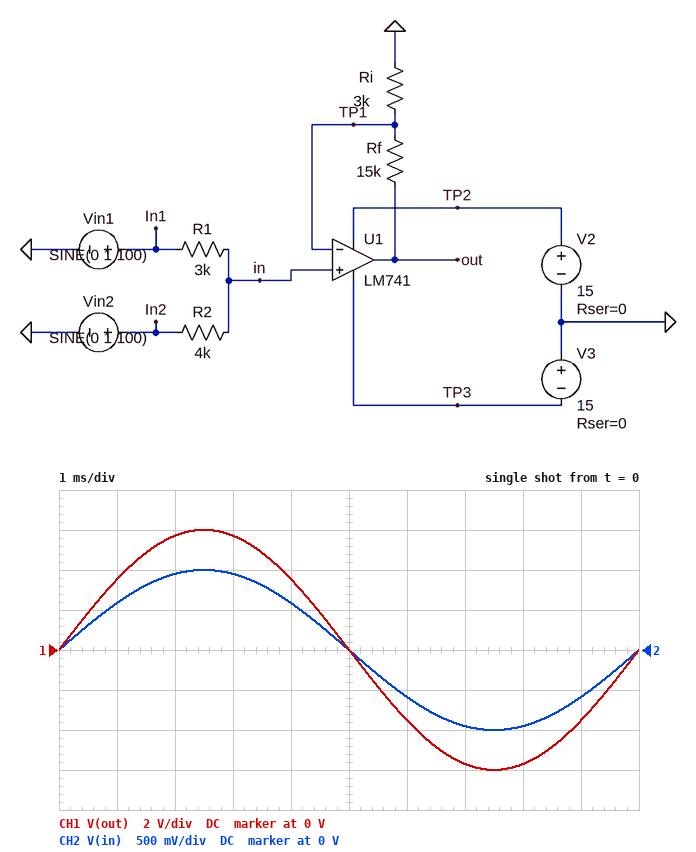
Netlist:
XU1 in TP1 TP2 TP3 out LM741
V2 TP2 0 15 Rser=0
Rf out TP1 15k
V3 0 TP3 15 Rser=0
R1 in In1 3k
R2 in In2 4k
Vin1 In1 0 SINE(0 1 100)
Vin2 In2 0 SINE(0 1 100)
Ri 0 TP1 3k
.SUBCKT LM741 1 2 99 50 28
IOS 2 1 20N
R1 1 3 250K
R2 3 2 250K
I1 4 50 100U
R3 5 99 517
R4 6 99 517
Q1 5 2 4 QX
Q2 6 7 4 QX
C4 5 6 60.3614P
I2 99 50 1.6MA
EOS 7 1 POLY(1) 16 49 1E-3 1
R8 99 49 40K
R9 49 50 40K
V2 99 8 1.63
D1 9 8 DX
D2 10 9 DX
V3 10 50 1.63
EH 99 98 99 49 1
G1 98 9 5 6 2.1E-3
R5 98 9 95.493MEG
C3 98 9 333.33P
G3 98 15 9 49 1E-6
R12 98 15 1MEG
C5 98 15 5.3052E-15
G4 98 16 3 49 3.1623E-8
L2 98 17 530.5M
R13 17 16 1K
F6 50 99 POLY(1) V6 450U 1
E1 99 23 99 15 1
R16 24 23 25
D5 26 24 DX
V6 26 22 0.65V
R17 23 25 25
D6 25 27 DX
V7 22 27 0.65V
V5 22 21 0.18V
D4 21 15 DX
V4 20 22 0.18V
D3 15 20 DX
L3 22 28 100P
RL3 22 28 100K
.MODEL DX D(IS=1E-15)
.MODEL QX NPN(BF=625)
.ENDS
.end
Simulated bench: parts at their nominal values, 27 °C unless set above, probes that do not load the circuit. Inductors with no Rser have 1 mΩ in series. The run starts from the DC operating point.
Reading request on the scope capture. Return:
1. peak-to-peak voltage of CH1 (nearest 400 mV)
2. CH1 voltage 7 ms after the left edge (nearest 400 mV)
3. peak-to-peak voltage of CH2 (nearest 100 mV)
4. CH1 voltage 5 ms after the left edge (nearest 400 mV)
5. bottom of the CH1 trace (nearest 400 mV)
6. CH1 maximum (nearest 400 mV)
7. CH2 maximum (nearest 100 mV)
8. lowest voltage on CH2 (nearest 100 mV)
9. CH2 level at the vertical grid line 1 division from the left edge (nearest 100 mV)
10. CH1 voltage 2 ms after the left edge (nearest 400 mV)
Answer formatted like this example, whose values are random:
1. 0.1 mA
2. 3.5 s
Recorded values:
1. 12.0 V
2. -5.6 V
3. 2.0 V
4. 0 V
5. -6.0 V
6. 6.0 V
7. 1.0 V
8. -1.0 V
9. 600 mV
10. 5.6 V
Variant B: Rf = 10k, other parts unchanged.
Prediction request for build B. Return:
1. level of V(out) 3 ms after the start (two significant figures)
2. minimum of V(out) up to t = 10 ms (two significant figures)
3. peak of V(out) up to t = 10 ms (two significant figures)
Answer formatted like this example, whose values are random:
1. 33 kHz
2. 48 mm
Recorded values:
1. 4.1 V
2. -4.3 V
3. 4.3 V
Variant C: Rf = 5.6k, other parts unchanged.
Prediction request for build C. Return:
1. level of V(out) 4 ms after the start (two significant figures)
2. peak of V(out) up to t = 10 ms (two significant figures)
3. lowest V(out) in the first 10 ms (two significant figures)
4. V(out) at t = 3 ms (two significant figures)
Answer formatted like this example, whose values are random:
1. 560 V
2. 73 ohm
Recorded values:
1. 1.7 V
2. 2.9 V
3. -2.9 V
4. 2.7 V
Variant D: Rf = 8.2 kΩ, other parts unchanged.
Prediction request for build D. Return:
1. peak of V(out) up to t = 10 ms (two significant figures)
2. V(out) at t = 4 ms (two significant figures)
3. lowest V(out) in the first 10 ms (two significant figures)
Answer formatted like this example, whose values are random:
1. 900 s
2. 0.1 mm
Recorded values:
1. 3.7 V
2. 2.2 V
3. -3.7 V
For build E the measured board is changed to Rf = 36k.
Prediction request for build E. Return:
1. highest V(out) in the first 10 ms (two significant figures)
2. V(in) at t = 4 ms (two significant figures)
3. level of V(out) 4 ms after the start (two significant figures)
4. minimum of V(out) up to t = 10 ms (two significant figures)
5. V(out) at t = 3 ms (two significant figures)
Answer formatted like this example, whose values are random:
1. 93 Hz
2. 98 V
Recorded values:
1. 13 V
2. 590 mV
3. 7.7 V
4. -13 V
5. 12 V
